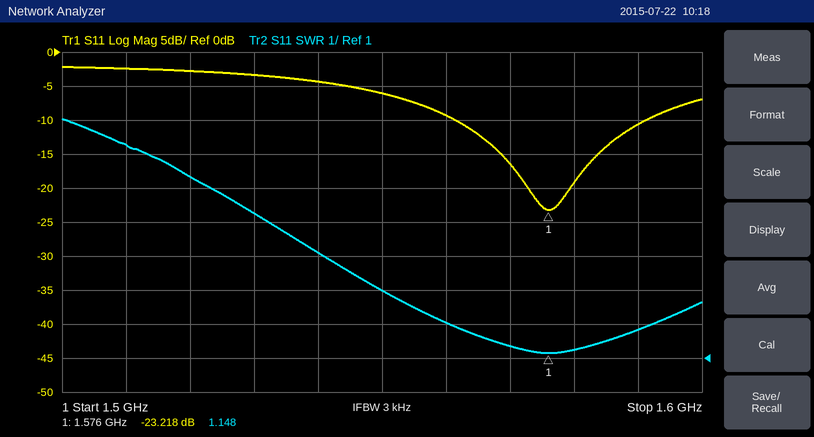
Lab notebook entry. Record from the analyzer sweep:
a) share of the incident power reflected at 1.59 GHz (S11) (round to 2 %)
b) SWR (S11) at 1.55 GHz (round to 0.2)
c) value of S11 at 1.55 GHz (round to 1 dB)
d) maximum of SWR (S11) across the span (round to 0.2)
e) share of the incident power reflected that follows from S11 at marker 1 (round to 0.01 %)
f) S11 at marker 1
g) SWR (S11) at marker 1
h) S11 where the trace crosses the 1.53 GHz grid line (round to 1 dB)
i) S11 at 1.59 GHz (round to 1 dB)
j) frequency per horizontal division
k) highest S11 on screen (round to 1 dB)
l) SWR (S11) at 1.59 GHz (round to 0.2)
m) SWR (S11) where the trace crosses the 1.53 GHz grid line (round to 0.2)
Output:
8 %
3.0
-6 dB
8.0
0.48 %
-23.218 dB
1.148
-3 dB
-11 dB
10 MHz
-2 dB
1.8
5.2
